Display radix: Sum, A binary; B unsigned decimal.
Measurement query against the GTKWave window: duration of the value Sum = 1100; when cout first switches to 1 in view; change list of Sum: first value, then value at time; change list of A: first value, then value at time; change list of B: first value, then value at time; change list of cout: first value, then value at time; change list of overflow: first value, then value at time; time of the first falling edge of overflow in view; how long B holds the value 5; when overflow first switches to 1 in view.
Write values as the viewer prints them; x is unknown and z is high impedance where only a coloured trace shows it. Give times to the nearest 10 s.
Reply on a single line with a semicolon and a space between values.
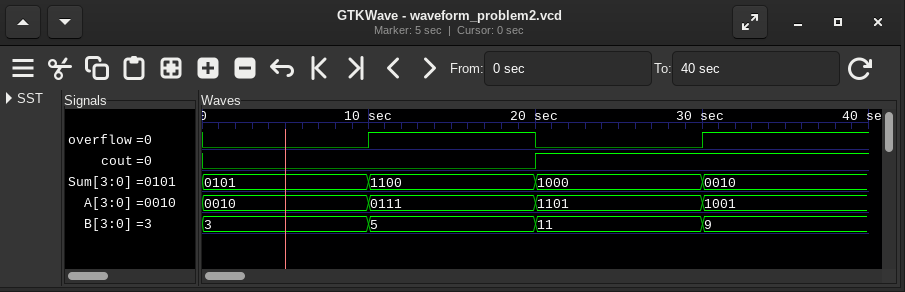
10 s; 20 s; 0101, 1100 at 10 s, 1000 at 20 s, 0010 at 30 s; 0010, 0111 at 10 s, 1101 at 20 s, 1001 at 30 s; 3, 5 at 10 s, 11 at 20 s, 9 at 30 s; 0, 1 at 20 s; 0, 1 at 10 s, 0 at 20 s, 1 at 30 s; 20 s; 10 s; 10 s
